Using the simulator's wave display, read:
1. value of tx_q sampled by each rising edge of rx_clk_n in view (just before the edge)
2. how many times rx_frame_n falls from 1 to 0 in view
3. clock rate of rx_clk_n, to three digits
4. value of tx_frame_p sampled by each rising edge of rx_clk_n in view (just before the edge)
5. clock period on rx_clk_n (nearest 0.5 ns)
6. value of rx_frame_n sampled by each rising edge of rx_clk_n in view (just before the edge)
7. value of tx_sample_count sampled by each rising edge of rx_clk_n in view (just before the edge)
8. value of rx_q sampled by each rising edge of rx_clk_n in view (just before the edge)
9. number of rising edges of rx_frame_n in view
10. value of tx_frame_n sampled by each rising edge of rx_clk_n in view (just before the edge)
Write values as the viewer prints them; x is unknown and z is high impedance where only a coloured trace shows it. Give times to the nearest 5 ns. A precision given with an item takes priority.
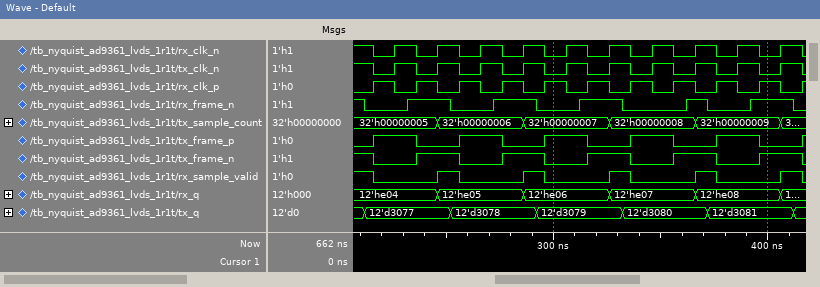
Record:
12'd3077, 12'd3077, 12'd3078, 12'd3078, 12'd3079, 12'd3079, 12'd3080, 12'd3080, 12'd3081, 12'd3081
6
50.0 MHz
1 0 1 0 1 0 1 0 1 0
20 ns
0 1 0 1 0 1 0 1 0 1
32'h00000005, 32'h00000005, 32'h00000006, 32'h00000006, 32'h00000007, 32'h00000007, 32'h00000008, 32'h00000008, 32'h00000009, 32'h00000009
12'he04, 12'he04, 12'he05, 12'he05, 12'he06, 12'he06, 12'he07, 12'he07, 12'he08, 12'he08
5
0 1 0 1 0 1 0 1 0 1
